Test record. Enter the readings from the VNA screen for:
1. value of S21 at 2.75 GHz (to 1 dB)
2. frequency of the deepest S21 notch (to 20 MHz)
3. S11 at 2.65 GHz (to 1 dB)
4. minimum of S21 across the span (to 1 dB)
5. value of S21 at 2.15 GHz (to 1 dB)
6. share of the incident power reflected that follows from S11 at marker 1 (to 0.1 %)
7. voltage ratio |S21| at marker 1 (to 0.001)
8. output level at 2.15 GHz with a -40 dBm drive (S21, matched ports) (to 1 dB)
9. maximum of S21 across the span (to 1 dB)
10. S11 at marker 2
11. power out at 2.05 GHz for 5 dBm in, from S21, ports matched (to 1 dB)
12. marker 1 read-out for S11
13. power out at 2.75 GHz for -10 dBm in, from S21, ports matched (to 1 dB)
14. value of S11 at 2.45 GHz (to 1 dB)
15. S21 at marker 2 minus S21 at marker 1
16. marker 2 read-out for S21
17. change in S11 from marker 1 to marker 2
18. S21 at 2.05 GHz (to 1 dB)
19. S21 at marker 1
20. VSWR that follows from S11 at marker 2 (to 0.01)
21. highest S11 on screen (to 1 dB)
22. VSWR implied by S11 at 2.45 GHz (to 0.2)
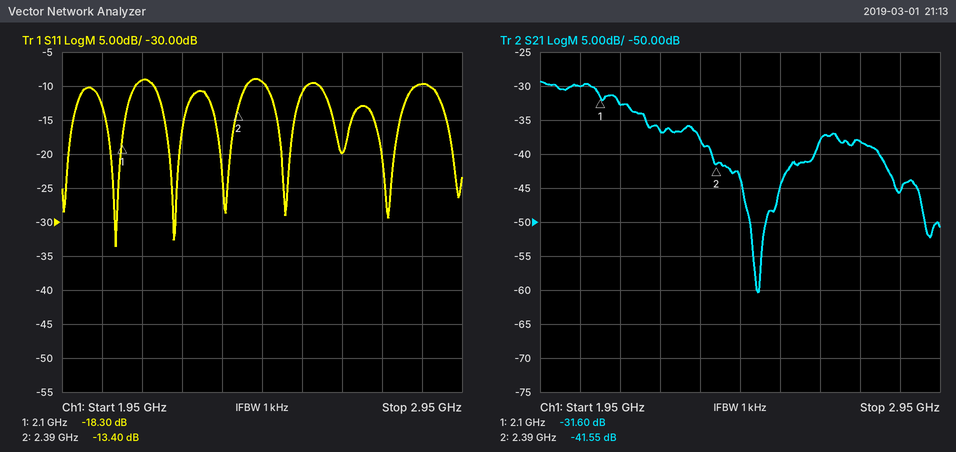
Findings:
-38 dB
2.50 GHz
-20 dB
-60 dB
-33 dB
1.5 %
0.026
-73 dBm
-29 dB
-13.40 dB
-25 dBm
-18.30 dB
-48 dBm
-9 dB
-9.95 dB
-41.55 dB
4.90 dB
-30 dB
-31.60 dB
1.54
-9 dB
2.0
